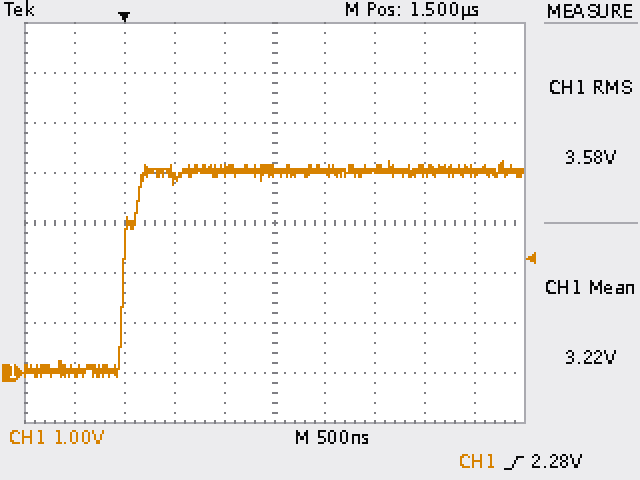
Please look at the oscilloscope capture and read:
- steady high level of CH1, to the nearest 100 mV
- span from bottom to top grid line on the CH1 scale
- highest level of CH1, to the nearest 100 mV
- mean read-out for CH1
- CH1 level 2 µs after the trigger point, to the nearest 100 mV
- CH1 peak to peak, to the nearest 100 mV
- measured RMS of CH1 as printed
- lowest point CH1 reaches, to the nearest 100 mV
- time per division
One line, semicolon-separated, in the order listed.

4.0 V; 8 V; 4.2 V; 3.22 V; 4.0 V; 4.3 V; 3.58 V; -100 mV; 500 ns
